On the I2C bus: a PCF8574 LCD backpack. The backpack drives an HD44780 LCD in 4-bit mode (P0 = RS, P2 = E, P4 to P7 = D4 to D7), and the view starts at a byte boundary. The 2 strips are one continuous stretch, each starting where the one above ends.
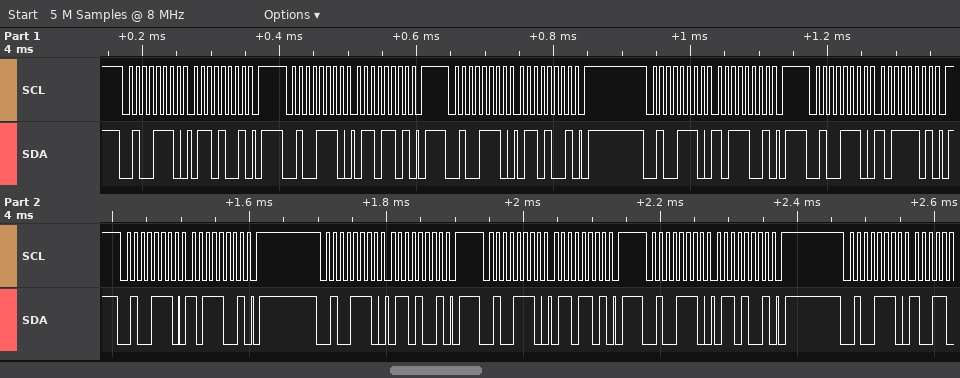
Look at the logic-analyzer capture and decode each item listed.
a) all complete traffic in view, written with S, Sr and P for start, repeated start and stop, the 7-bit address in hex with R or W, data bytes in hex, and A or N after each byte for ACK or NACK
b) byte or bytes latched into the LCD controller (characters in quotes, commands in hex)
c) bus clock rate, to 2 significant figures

S 27W A 69 A P S 27W A 6D A P S 27W A 69 A P S 27W A B9 A P S 27W A BD A P S 27W A B9 A P S 27W A 69 A P S 27W A 6D A P S 27W A 69 A P S 27W A
'k'
100 kHz
